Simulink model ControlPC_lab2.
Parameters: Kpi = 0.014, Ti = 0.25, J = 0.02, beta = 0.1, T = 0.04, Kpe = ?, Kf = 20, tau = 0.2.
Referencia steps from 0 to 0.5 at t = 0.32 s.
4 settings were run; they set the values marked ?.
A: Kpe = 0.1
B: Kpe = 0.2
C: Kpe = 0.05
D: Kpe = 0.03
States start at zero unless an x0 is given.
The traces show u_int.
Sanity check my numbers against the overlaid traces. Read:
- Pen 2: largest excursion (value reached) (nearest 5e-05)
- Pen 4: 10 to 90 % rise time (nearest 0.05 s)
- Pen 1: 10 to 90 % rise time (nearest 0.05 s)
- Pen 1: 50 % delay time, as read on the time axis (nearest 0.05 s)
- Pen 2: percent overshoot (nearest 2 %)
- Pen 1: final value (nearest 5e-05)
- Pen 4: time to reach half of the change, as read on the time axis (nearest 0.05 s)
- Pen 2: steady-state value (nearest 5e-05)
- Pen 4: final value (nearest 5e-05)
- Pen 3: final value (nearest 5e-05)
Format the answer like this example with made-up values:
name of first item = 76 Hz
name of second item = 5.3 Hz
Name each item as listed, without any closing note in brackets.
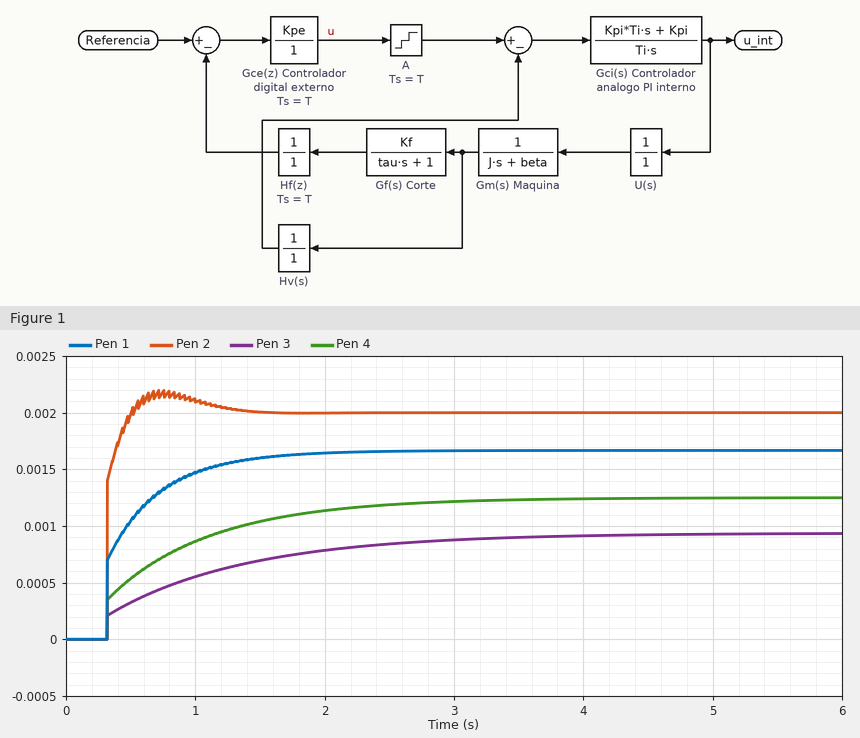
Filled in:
Pen 2: largest excursion (value reached) = 0.00220
Pen 4: 10 to 90 % rise time = 1.60 s
Pen 1: 10 to 90 % rise time = 0.75 s
Pen 1: 50 % delay time, as read on the time axis = 0.40 s
Pen 2: percent overshoot = 10 %
Pen 1: final value = 0.00165
Pen 4: time to reach half of the change, as read on the time axis = 0.60 s
Pen 2: steady-state value = 0.00200
Pen 4: final value = 0.00125
Pen 3: final value = 0.00095
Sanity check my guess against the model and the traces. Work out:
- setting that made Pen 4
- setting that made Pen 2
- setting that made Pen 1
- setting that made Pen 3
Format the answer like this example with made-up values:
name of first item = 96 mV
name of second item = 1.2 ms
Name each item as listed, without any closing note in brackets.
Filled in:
setting that made Pen 4 = C
setting that made Pen 2 = B
setting that made Pen 1 = A
setting that made Pen 3 = D
